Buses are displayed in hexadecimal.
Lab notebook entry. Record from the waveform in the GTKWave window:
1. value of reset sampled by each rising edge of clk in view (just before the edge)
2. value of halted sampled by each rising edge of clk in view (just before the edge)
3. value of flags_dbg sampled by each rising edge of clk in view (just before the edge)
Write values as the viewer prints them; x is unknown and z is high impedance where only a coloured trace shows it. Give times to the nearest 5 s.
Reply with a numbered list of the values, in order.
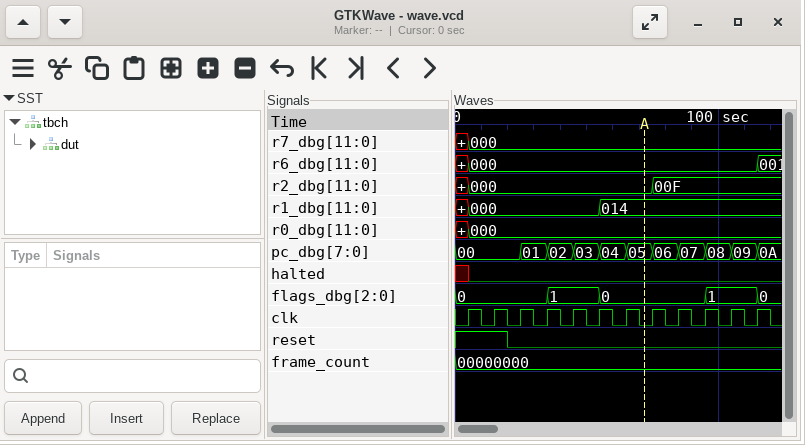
1. 1 1 0 0 0 0 0 0 0 0 0 0
2. x 0 0 0 0 0 0 0 0 0 0 0
3. 0, 0, 0, 0, 1, 1, 0, 0, 0, 0, 1, 1
